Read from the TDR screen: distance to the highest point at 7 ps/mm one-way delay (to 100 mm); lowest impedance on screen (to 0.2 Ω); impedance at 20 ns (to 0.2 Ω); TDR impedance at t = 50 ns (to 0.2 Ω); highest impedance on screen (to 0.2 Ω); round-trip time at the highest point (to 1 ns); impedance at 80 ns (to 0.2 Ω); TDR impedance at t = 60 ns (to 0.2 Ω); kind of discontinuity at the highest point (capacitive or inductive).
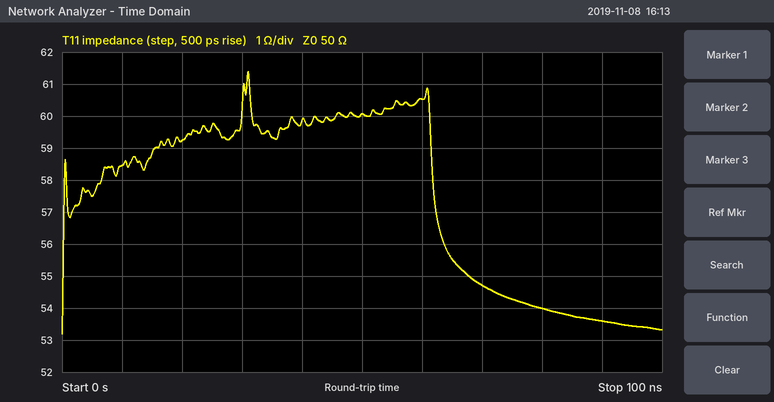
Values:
2.2 m
53.2 Ω
59.2 Ω
60.0 Ω
61.4 Ω
31 ns
54.0 Ω
60.6 Ω
inductive
